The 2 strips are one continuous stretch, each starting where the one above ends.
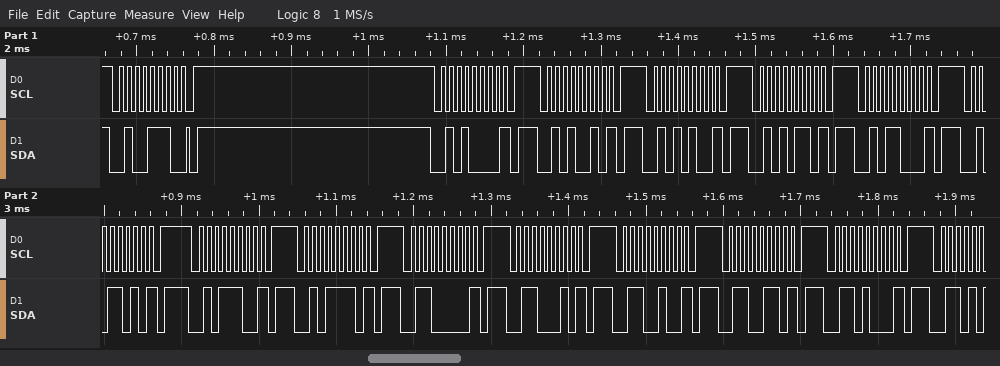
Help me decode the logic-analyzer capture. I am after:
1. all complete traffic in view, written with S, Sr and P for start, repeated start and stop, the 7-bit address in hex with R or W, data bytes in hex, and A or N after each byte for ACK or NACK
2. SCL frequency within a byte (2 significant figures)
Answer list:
S 27W A P S 28W N P S 29W N P S 2AW N P S 2BW N P S 2CW N P S 2DW N P S 2EW N P S 2FW N P S 30W N P S 31W N P S 32W N P S 33W N P S 34W N P
100 kHz
